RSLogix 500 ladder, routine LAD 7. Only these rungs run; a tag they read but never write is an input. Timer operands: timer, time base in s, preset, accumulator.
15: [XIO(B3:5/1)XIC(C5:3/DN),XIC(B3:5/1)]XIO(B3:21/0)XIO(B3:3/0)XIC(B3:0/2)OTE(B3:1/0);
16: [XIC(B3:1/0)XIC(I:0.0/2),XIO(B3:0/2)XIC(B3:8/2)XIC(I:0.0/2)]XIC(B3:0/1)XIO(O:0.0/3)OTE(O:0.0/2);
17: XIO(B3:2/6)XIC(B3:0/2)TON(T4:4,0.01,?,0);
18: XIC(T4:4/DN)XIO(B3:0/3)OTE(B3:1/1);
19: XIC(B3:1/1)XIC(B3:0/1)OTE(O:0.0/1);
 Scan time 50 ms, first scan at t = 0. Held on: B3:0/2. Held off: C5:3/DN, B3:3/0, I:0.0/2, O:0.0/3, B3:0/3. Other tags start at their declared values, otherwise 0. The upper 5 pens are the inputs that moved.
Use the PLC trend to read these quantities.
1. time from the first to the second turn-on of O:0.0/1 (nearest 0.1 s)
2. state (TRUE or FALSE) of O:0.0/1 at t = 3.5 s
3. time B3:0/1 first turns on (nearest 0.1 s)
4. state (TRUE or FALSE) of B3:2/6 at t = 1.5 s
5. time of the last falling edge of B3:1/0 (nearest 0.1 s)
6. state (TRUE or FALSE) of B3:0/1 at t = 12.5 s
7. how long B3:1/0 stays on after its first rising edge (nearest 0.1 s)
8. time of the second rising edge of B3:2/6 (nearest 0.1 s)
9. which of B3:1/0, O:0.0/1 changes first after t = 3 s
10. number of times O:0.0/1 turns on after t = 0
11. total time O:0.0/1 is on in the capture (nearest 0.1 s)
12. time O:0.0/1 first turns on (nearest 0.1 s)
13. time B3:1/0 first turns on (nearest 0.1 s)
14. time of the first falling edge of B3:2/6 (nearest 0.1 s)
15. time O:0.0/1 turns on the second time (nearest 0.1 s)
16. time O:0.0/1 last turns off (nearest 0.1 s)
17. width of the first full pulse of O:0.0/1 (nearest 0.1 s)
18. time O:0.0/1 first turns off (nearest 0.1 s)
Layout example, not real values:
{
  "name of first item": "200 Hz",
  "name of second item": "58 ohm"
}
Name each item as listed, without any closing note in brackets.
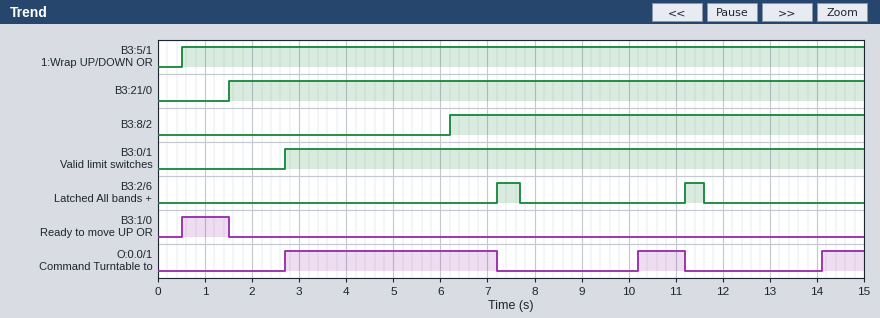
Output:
{
  "time from the first to the second turn-on of O:0.0/1": "7.5 s",
  "state (TRUE or FALSE) of O:0.0/1 at t = 3.5 s": "TRUE",
  "time B3:0/1 first turns on": "2.7 s",
  "state (TRUE or FALSE) of B3:2/6 at t = 1.5 s": "FALSE",
  "time of the last falling edge of B3:1/0": "1.5 s",
  "state (TRUE or FALSE) of B3:0/1 at t = 12.5 s": "TRUE",
  "how long B3:1/0 stays on after its first rising edge": "1.0 s",
  "time of the second rising edge of B3:2/6": "11.2 s",
  "which of B3:1/0, O:0.0/1 changes first after t = 3 s": "O:0.0/1",
  "number of times O:0.0/1 turns on after t = 0": "3",
  "total time O:0.0/1 is on in the capture": "6.4 s",
  "time O:0.0/1 first turns on": "2.7 s",
  "time B3:1/0 first turns on": "0.5 s",
  "time of the first falling edge of B3:2/6": "7.7 s",
  "time O:0.0/1 turns on the second time": "10.2 s",
  "time O:0.0/1 last turns off": "11.2 s",
  "width of the first full pulse of O:0.0/1": "4.5 s",
  "time O:0.0/1 first turns off": "7.2 s"
}
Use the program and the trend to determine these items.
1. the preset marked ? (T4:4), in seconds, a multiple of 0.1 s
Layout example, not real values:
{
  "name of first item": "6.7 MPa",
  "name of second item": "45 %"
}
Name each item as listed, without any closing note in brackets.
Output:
{
  "the preset marked ? (T4:4), in seconds, a multiple of 0.1 s": "2.5 s"
}
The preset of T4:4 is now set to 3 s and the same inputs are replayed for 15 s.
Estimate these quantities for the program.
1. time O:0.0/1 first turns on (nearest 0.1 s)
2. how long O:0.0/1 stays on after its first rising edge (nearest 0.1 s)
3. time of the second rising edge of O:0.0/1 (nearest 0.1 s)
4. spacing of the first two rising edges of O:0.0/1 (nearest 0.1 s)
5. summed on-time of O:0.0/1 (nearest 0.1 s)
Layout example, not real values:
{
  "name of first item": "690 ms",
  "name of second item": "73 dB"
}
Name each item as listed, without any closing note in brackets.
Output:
{
  "time O:0.0/1 first turns on": "3.0 s",
  "how long O:0.0/1 stays on after its first rising edge": "4.2 s",
  "time of the second rising edge of O:0.0/1": "10.7 s",
  "spacing of the first two rising edges of O:0.0/1": "7.7 s",
  "summed on-time of O:0.0/1": "5.1 s"
}
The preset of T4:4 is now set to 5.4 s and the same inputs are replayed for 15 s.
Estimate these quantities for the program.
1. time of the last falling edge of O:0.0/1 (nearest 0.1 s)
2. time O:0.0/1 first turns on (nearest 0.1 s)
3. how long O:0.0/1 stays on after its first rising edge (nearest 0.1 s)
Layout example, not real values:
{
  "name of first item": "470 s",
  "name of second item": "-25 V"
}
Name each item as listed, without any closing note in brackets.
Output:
{
  "time of the last falling edge of O:0.0/1": "7.2 s",
  "time O:0.0/1 first turns on": "5.4 s",
  "how long O:0.0/1 stays on after its first rising edge": "1.8 s"
}
